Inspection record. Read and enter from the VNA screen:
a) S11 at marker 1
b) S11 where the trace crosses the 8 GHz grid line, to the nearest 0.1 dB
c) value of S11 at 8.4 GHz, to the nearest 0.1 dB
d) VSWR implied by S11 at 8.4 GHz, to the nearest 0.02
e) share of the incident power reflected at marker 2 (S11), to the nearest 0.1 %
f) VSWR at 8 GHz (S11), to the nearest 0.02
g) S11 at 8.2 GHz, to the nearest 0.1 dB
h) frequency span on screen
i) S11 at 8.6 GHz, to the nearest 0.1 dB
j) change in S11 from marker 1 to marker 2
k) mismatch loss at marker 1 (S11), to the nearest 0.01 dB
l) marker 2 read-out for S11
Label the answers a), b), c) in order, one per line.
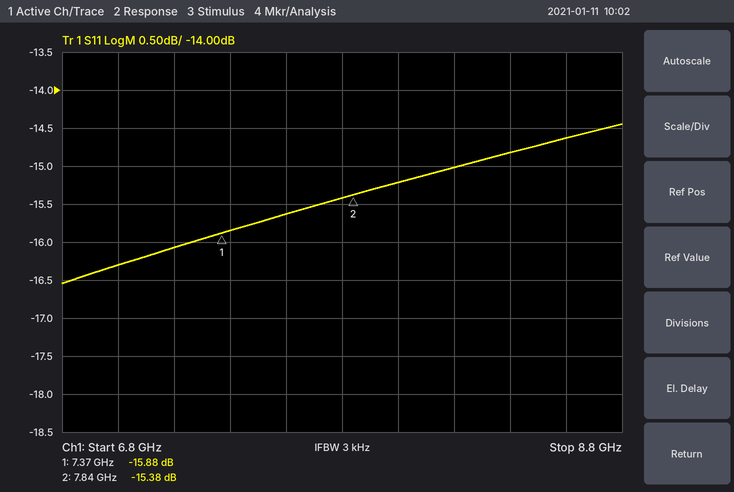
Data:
a) -15.88 dB
b) -15.2 dB
c) -14.8 dB
d) 1.44
e) 2.9 %
f) 1.42
g) -15.0 dB
h) 2 GHz
i) -14.6 dB
j) 0.50 dB
k) 0.11 dB
l) -15.38 dB
